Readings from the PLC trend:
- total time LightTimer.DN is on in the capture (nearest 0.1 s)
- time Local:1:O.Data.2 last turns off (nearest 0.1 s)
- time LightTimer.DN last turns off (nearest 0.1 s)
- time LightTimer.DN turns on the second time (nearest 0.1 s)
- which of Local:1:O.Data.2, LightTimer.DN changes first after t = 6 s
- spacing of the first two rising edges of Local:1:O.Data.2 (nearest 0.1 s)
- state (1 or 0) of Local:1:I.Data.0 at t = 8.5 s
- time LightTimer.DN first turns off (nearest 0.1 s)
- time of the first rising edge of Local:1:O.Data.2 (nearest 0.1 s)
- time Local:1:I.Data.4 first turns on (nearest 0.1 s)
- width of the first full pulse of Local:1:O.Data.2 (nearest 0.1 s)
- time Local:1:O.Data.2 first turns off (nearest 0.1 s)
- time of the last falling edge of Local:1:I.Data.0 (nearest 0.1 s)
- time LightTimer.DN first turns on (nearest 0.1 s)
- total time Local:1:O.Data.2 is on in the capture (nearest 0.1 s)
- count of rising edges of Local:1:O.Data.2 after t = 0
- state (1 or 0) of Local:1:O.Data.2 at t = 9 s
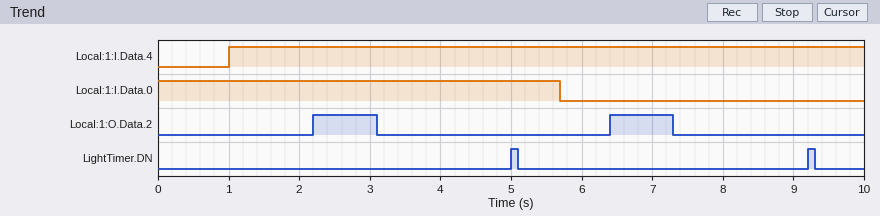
0.2 s
7.3 s
9.3 s
9.2 s
Local:1:O.Data.2
4.2 s
0
5.1 s
2.2 s
1.0 s
0.9 s
3.1 s
5.7 s
5.0 s
1.8 s
2
0
